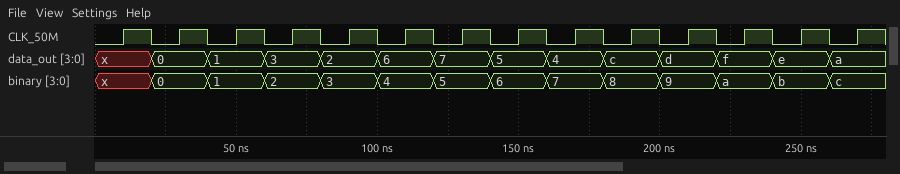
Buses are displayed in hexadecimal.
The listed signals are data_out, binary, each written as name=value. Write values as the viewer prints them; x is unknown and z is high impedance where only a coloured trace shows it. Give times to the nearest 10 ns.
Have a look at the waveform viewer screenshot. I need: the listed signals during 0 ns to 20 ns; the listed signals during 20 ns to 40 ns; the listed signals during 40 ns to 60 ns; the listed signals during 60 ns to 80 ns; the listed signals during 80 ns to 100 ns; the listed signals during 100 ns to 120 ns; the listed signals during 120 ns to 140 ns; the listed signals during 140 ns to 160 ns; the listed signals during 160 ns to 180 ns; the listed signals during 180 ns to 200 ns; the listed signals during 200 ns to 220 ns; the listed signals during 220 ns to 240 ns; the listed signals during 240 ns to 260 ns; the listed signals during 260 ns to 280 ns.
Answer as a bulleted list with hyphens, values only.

- data_out=x, binary=x
- data_out=0, binary=0
- data_out=1, binary=1
- data_out=3, binary=2
- data_out=2, binary=3
- data_out=6, binary=4
- data_out=7, binary=5
- data_out=5, binary=6
- data_out=4, binary=7
- data_out=c, binary=8
- data_out=d, binary=9
- data_out=f, binary=a
- data_out=e, binary=b
- data_out=a, binary=c
